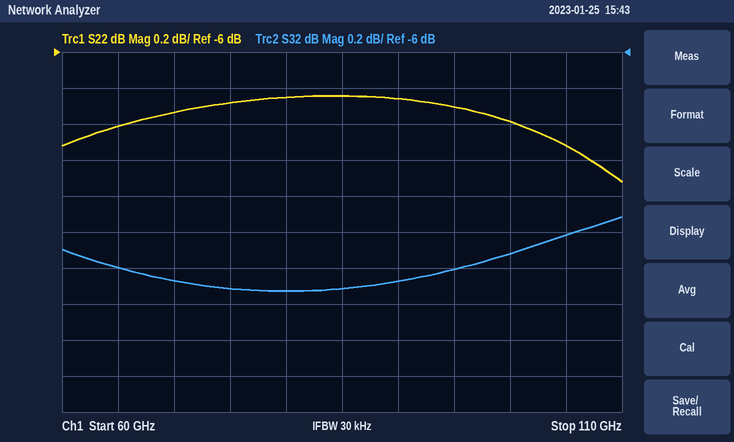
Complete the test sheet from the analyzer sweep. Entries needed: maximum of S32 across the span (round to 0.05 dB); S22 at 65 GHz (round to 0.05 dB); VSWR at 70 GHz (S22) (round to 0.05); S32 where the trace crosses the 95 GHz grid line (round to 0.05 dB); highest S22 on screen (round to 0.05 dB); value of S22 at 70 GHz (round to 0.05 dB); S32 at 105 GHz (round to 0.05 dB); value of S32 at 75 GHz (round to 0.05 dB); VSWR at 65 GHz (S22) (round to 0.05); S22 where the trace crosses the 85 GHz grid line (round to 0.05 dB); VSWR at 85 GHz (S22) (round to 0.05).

-6.90 dB
-6.40 dB
2.85
-7.20 dB
-6.25 dB
-6.35 dB
-7.00 dB
-7.30 dB
2.85
-6.25 dB
2.90
